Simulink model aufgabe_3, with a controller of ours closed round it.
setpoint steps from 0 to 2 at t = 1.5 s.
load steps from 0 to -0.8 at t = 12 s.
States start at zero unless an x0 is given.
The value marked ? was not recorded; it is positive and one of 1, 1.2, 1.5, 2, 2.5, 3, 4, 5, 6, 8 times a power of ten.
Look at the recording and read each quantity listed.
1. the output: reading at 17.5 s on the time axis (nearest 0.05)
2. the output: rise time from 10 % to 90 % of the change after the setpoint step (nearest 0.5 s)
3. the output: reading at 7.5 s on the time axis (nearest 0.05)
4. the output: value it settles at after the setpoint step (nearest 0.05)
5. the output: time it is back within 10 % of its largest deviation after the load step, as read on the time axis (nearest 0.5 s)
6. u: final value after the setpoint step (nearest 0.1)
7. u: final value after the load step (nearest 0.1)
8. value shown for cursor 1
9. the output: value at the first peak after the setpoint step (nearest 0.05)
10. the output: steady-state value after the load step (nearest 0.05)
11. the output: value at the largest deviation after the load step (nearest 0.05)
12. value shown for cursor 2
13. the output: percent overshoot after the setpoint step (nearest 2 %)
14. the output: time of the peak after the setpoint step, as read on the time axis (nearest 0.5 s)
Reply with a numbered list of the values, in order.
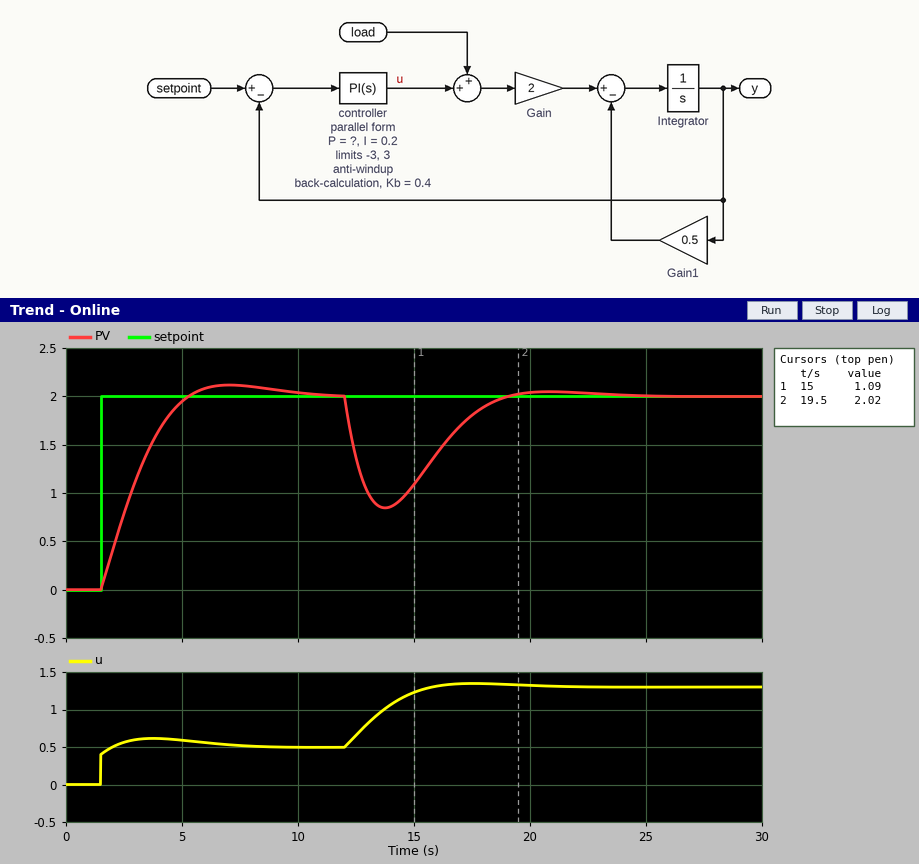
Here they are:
1. 1.80
2. 2.5 s
3. 2.10
4. 2.00
5. 18.0 s
6. 0.5
7. 1.3
8. 1.09
9. 2.10
10. 2.00
11. 0.85
12. 2.02
13. 6 %
14. 7.0 s
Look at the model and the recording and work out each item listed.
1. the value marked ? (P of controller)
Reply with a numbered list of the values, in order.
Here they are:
1. 0.2
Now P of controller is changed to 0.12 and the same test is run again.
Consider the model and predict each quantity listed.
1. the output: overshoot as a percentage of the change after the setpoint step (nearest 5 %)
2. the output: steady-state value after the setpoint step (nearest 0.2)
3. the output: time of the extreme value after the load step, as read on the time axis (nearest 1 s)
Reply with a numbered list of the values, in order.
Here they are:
1. 10 %
2. 2.0
3. 14 s
